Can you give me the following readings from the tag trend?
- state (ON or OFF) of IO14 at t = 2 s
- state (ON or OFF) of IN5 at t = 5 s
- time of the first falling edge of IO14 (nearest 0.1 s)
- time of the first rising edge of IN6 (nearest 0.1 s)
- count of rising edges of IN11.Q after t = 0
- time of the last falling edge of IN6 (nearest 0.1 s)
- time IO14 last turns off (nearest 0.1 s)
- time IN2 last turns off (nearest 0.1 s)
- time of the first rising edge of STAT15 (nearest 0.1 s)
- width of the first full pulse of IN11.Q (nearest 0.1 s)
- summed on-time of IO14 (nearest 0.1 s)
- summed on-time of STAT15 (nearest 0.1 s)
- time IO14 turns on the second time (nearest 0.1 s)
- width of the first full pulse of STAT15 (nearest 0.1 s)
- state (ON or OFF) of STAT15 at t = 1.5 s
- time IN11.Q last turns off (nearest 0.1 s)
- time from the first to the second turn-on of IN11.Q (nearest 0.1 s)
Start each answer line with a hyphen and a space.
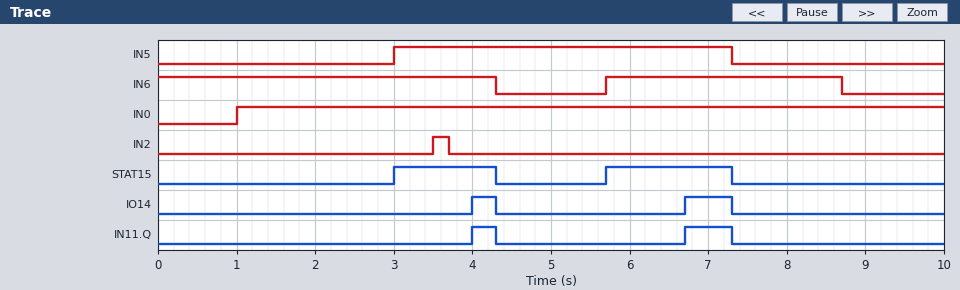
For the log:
- OFF
- ON
- 4.3 s
- 5.7 s
- 2
- 8.7 s
- 7.3 s
- 3.7 s
- 3.0 s
- 0.3 s
- 0.9 s
- 2.9 s
- 6.7 s
- 1.3 s
- OFF
- 7.3 s
- 2.7 s
